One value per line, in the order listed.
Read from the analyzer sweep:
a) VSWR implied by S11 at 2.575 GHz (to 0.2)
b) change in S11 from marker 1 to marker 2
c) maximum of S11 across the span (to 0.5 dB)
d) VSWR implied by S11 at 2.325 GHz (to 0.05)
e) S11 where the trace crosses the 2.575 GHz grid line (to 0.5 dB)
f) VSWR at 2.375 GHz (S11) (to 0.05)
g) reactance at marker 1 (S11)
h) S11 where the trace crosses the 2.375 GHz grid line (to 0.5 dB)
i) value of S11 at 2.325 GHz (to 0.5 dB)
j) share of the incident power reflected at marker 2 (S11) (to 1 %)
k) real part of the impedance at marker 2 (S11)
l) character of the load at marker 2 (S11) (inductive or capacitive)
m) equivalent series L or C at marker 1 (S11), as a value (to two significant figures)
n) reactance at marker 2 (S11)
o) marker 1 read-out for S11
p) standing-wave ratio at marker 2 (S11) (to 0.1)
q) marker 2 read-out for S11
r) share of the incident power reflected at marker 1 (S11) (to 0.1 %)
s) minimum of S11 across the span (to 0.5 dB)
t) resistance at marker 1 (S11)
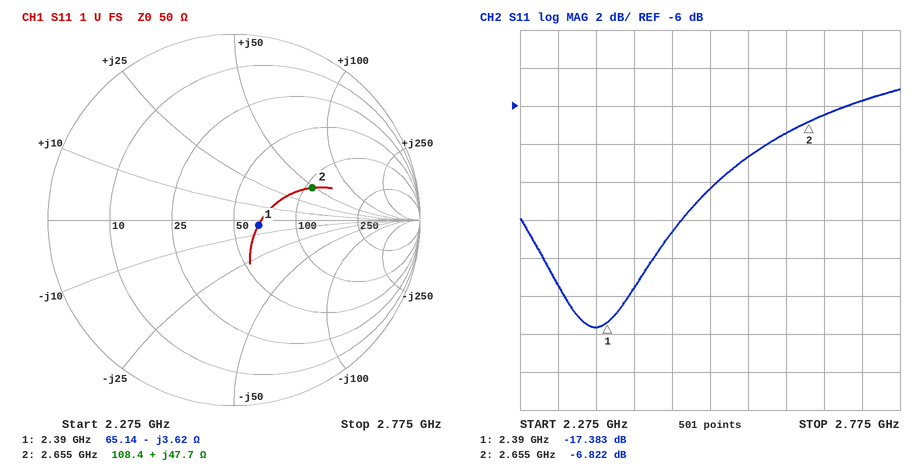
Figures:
2.2
10.561 dB
-5.0 dB
1.40
-8.5 dB
1.30
-3.62 Ω
-17.5 dB
-15.5 dB
21 %
108.4 Ω
inductive
18 pF
+47.7 Ω
-17.383 dB
2.7
-6.822 dB
1.8 %
-17.5 dB
65.14 Ω
